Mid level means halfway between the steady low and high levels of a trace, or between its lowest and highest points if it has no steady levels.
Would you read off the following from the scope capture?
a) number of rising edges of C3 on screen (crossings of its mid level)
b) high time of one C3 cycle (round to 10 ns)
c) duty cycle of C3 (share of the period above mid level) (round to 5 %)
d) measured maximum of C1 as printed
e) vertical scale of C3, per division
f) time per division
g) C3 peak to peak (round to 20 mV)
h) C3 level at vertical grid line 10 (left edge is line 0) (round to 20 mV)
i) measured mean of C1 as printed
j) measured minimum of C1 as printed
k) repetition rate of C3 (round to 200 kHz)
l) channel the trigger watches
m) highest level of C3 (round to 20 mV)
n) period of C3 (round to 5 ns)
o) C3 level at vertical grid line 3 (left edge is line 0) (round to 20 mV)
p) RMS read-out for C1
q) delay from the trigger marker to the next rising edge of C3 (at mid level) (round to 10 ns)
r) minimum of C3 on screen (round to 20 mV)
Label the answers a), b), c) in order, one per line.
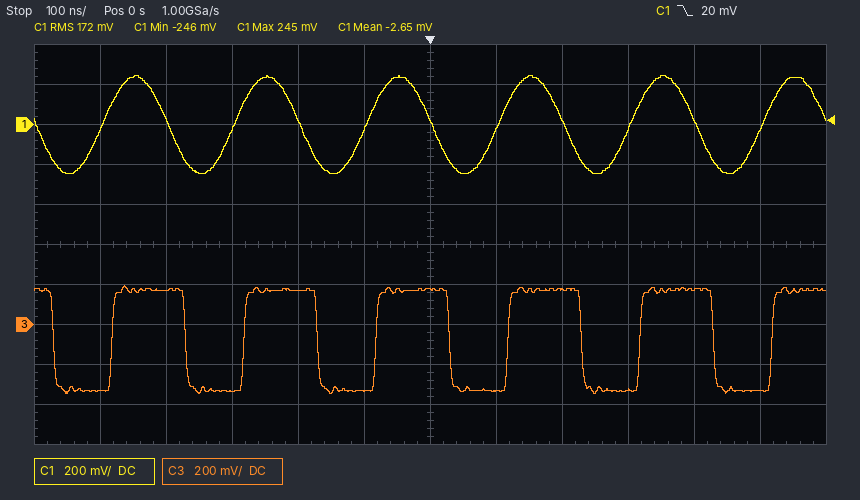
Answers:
a) 6
b) 110 ns
c) 55 %
d) 245 mV
e) 200 mV
f) 100 ns
g) 540 mV
h) 180 mV
i) -2.65 mV
j) -246 mV
k) 5.0 MHz
l) C1
m) 200 mV
n) 200 ns
o) -340 mV
p) 172 mV
q) 120 ns
r) -340 mV
